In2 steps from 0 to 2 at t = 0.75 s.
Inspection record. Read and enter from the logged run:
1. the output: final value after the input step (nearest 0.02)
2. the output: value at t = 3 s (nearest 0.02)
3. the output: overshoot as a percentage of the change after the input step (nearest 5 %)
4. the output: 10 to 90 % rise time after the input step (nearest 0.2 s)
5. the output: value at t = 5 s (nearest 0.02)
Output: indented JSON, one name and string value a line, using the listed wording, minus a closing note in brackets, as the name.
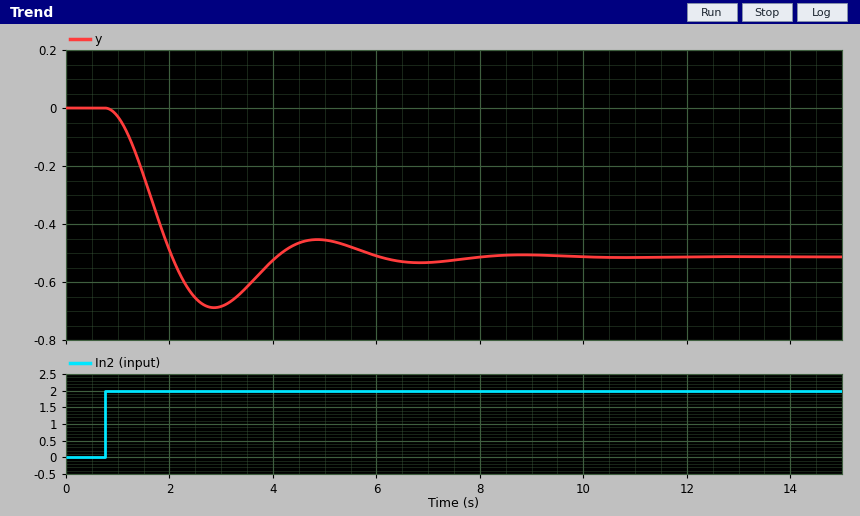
{
  "the output: final value after the input step": "-0.52",
  "the output: value at t = 3 s": "-0.68",
  "the output: overshoot as a percentage of the change after the input step": "35 %",
  "the output: 10 to 90 % rise time after the input step": "0.8 s",
  "the output: value at t = 5 s": "-0.46"
}
